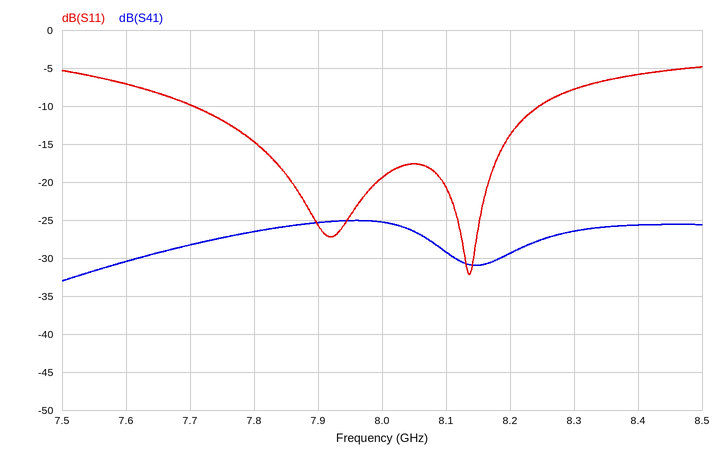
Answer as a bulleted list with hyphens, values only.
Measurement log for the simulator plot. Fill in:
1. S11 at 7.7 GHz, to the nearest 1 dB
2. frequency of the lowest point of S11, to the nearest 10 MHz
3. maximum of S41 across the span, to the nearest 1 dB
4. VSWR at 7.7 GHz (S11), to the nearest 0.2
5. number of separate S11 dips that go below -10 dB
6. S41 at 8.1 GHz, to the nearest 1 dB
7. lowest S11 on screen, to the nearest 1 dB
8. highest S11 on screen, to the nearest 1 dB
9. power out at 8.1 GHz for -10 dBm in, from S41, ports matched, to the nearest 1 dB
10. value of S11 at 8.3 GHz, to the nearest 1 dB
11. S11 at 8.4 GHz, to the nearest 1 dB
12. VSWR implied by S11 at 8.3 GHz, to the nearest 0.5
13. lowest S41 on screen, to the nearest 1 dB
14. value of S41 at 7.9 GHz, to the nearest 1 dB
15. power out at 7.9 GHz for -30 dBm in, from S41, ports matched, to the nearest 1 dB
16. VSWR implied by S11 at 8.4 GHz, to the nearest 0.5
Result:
- -10 dB
- 8.14 GHz
- -25 dB
- 2.0
- 2
- -29 dB
- -32 dB
- -5 dB
- -39 dBm
- -8 dB
- -6 dB
- 2.5
- -33 dB
- -25 dB
- -55 dBm
- 3.0
